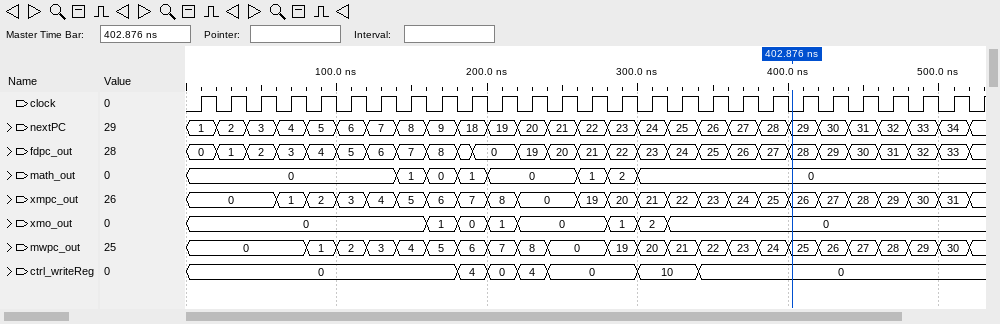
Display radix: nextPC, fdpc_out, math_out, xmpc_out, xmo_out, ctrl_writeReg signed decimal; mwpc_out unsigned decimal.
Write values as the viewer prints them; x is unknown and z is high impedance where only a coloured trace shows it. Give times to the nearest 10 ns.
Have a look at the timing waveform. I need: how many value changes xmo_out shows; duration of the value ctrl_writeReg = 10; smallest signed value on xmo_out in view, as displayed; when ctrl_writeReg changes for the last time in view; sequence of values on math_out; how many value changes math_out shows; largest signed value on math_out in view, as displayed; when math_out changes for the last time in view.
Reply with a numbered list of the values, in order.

1. 7
2. 40 ns
3. 0
4. 340 ns
5. 0, 1, 0, 1, 0, 1, 2, 0
6. 7
7. 2
8. 300 ns
